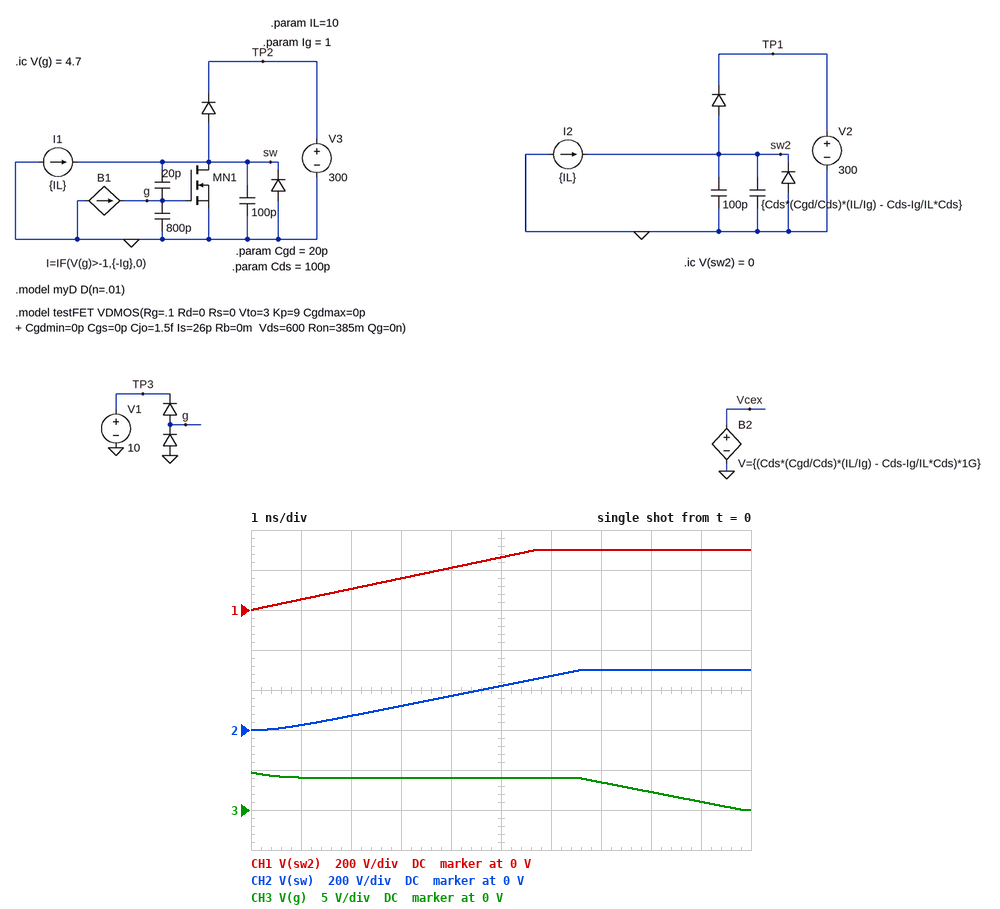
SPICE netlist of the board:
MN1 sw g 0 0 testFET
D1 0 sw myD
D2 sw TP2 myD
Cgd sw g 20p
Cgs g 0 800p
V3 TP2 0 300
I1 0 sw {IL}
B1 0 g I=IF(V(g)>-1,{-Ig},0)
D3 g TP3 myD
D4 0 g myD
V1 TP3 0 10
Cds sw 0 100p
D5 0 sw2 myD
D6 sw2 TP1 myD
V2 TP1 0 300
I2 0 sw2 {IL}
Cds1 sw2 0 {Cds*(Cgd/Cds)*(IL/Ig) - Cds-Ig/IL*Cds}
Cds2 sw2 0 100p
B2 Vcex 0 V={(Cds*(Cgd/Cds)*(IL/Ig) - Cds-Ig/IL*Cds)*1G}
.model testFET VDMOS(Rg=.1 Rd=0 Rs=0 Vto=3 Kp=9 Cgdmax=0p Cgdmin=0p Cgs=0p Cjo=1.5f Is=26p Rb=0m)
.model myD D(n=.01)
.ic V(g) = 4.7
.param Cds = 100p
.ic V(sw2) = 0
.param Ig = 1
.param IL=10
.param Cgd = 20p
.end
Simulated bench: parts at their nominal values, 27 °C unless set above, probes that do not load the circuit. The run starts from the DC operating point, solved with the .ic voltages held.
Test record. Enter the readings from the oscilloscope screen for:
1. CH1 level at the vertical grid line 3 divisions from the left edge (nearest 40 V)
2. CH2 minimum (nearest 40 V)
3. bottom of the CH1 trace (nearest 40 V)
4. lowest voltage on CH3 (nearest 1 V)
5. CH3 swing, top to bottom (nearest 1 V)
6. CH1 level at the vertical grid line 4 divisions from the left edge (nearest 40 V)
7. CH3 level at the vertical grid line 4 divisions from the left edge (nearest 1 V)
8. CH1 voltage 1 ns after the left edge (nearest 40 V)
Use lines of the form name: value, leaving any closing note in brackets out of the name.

CH1 level at the vertical grid line 3 divisions from the left edge: 160 V
CH2 minimum: 0 V
bottom of the CH1 trace: 0 V
lowest voltage on CH3: 0 V
CH3 swing, top to bottom: 5 V
CH1 level at the vertical grid line 4 divisions from the left edge: 200 V
CH3 level at the vertical grid line 4 divisions from the left edge: 4 V
CH1 voltage 1 ns after the left edge: 40 V
